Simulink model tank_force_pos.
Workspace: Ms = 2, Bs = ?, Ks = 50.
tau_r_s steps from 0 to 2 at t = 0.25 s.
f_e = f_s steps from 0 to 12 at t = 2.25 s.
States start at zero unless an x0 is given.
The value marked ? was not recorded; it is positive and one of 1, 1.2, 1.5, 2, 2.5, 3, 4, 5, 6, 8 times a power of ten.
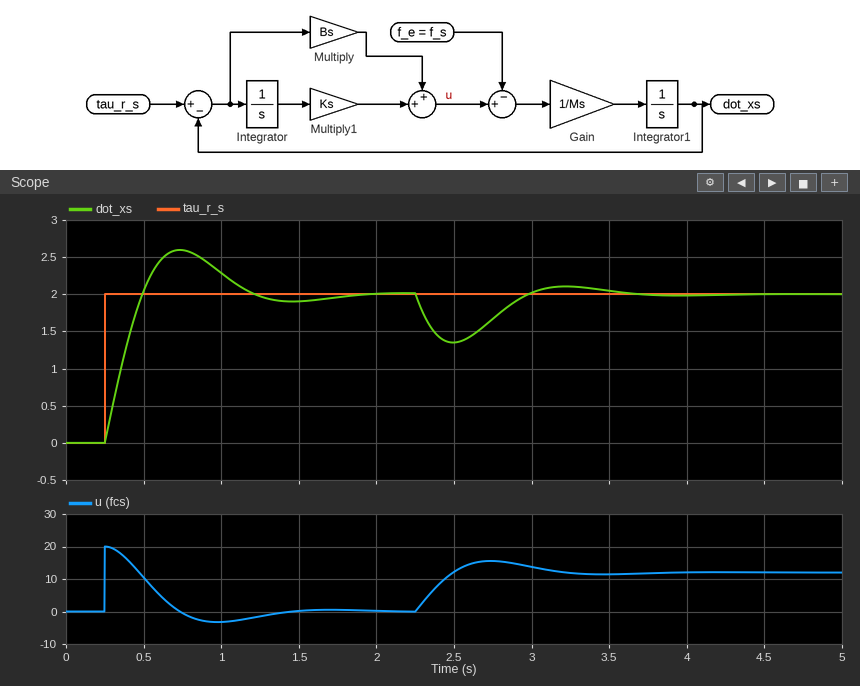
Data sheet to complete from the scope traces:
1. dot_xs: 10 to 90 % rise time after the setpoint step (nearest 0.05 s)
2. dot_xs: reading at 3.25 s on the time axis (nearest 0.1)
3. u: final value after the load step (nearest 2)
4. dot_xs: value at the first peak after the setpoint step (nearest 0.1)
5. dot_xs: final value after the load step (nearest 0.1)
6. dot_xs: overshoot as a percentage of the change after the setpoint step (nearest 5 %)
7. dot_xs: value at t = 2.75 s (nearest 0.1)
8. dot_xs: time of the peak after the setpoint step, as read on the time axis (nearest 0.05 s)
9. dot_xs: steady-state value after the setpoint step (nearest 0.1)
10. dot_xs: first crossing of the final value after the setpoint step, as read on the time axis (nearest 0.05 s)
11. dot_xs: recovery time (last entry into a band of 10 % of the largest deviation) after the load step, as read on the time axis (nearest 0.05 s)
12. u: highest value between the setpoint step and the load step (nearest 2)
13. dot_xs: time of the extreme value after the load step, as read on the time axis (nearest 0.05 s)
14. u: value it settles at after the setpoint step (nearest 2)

0.20 s
2.1
12
2.6
2.0
30 %
1.7
0.75 s
2.0
0.50 s
3.45 s
20
2.50 s
0
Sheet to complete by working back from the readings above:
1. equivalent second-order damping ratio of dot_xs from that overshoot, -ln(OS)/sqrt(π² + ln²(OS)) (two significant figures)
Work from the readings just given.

0.36
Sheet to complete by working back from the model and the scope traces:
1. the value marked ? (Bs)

10
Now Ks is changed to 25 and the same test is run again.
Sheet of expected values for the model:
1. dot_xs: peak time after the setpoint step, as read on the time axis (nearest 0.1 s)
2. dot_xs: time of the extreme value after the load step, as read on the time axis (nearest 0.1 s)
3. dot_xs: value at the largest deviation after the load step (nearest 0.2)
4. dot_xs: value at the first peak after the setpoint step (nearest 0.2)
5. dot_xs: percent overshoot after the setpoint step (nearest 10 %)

0.9 s
2.6 s
1.2
2.4
20 %
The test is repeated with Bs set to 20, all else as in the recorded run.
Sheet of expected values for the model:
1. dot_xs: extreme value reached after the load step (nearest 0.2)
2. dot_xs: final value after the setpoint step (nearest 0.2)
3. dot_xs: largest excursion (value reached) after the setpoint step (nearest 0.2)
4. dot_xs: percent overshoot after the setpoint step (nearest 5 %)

1.6
2.0
2.2
15 %
